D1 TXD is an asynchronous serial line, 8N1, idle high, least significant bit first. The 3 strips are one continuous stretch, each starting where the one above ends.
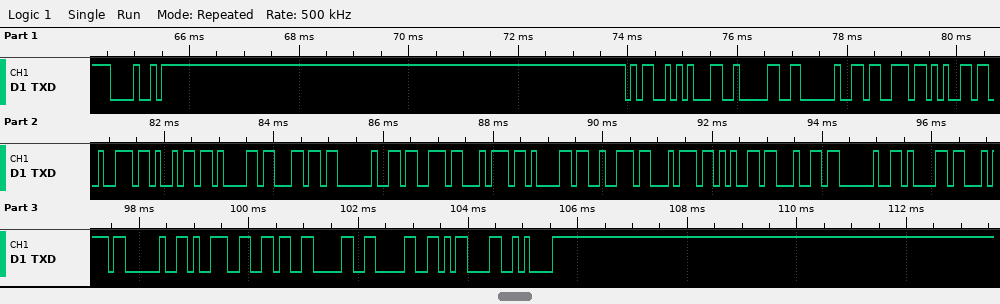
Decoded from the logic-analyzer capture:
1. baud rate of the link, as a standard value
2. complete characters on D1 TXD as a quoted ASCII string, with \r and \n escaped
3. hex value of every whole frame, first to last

9600 baud
"HM10 serial started at 9600\r\n"
48 4D 31 30 20 73 65 72 69 61 6C 20 73 74 61 72 74 65 64 20 61 74 20 39 36 30 30 0D 0A
